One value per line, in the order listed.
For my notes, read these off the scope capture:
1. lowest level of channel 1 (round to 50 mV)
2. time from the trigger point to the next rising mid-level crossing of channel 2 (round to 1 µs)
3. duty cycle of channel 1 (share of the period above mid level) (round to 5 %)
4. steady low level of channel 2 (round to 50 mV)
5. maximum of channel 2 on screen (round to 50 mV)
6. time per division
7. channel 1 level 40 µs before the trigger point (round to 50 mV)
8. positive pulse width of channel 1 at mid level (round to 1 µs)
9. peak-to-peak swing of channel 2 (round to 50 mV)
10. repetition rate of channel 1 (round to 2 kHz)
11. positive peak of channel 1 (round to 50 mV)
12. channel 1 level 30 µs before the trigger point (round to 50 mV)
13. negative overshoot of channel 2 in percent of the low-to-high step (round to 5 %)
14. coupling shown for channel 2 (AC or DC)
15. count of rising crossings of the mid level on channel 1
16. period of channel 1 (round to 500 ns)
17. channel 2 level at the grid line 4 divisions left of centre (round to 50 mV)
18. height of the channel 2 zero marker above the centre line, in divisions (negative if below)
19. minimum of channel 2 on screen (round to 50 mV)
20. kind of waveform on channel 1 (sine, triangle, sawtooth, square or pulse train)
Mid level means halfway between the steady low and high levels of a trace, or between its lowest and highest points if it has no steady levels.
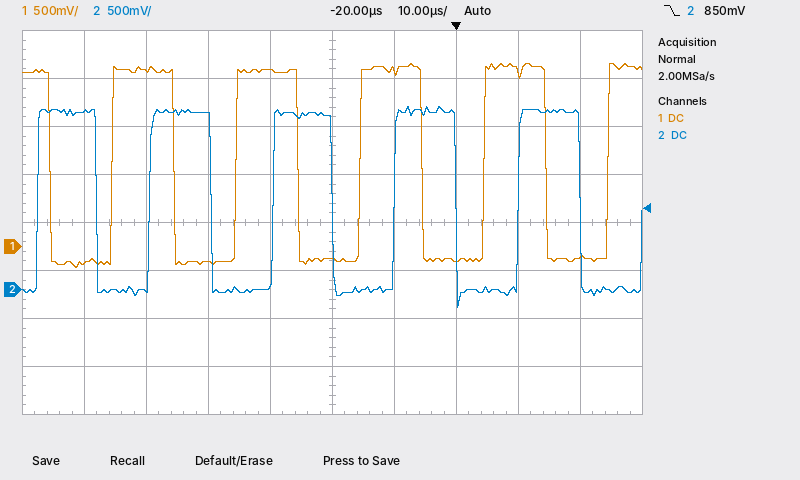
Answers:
-200 mV
10 µs
50 %
0 mV
1.90 V
10 µs
-150 mV
10 µs
2.10 V
50 kHz
1.90 V
1.85 V
10 %
DC
5
20.0 µs
1.85 V
-1.4 div
-200 mV
square
